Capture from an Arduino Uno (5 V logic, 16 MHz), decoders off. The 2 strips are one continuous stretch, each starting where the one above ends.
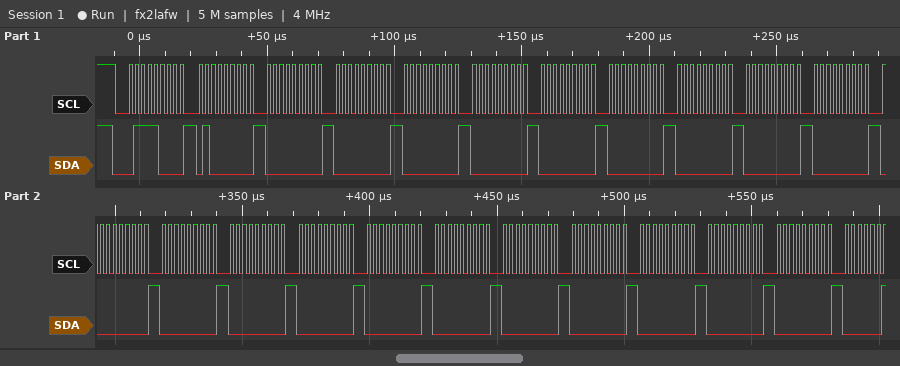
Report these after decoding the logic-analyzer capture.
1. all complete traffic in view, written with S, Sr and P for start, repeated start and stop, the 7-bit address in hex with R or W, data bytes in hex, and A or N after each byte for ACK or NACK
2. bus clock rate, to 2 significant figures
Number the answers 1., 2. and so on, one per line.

1. S 3CW A 40 A 00 A 00 A 00 A 00 A 00 A 00 A 00 A 00 A 00 A 00 A 00 A 00 A 00 A 00 A 00 A 00 A 00 A 00 A 00 A 00 A
2. 400 kHz
